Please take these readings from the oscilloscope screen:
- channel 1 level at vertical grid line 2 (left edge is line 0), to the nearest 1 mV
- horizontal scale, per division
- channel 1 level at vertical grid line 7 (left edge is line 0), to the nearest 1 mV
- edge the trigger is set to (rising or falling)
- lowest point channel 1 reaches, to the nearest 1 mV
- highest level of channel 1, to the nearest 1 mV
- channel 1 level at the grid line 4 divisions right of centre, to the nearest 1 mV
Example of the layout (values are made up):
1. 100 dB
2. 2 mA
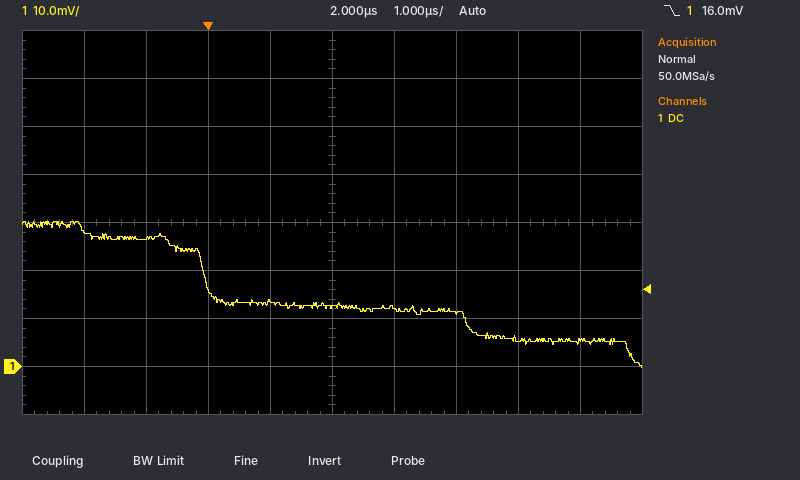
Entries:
1. 27 mV
2. 1 µs
3. 11 mV
4. falling
5. 0 mV
6. 30 mV
7. 5 mV
